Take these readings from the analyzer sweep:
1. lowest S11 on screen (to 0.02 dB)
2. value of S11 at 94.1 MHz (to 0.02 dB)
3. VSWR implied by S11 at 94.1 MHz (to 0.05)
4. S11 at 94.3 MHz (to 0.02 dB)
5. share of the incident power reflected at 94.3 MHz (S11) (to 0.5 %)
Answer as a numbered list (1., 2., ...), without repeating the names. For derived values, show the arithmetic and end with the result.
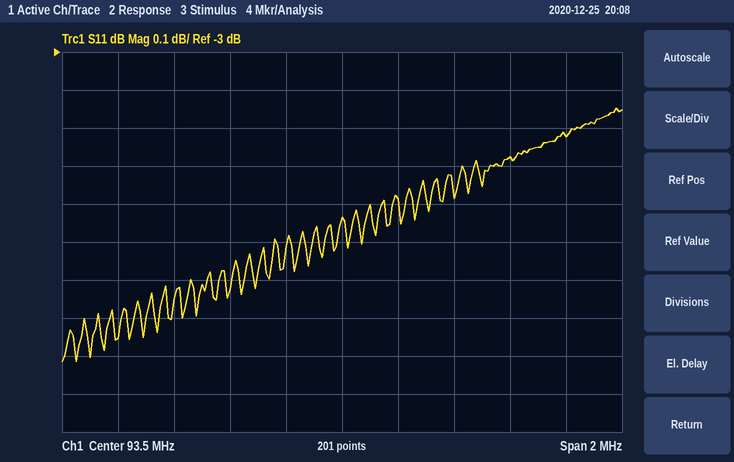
1. -3.82 dB
2. -3.28 dB
3. |Γ| = 10^(-3.28/20) = 0.6855; VSWR = (1 + 0.6855)/(1 − 0.6855) ≈ 5.36, so 5.35 to the nearest 0.05
4. -3.22 dB
5. 10^(-3.22/10) ≈ 47.6 %, so 47.5 % to the nearest 0.5 %
